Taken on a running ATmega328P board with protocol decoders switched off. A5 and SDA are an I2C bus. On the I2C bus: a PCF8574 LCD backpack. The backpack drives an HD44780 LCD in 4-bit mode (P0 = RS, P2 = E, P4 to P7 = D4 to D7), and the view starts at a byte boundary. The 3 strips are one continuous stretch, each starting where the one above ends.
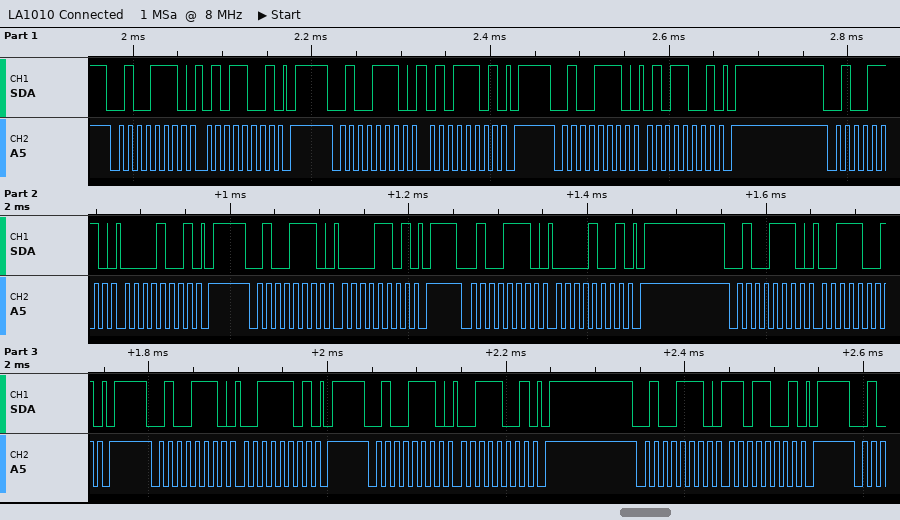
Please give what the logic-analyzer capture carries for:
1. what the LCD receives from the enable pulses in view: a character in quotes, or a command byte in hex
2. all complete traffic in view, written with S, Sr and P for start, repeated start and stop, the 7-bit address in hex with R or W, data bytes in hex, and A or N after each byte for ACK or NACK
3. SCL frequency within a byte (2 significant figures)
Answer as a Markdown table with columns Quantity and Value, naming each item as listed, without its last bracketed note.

| Quantity | Value |
|---|---|
| what the LCD receives from the enable pulses in view: a character in quotes, or a command byte in hex | 'P' |
| all complete traffic in view, written with S, Sr and P for start, repeated start and stop, the 7-bit address in hex with R or W, data bytes in hex, and A or N after each byte for ACK or NACK | S 27W A 59 A P S 27W A 5D A P S 27W A 59 A P S 27W A 09 A P S 27W A 0D A P S 27W A 09 A P S 27W A 39 A P S 27W A 3D A P S 27W A 39 A P S 27W A D9 A P |
| SCL frequency within a byte | 100 kHz |
